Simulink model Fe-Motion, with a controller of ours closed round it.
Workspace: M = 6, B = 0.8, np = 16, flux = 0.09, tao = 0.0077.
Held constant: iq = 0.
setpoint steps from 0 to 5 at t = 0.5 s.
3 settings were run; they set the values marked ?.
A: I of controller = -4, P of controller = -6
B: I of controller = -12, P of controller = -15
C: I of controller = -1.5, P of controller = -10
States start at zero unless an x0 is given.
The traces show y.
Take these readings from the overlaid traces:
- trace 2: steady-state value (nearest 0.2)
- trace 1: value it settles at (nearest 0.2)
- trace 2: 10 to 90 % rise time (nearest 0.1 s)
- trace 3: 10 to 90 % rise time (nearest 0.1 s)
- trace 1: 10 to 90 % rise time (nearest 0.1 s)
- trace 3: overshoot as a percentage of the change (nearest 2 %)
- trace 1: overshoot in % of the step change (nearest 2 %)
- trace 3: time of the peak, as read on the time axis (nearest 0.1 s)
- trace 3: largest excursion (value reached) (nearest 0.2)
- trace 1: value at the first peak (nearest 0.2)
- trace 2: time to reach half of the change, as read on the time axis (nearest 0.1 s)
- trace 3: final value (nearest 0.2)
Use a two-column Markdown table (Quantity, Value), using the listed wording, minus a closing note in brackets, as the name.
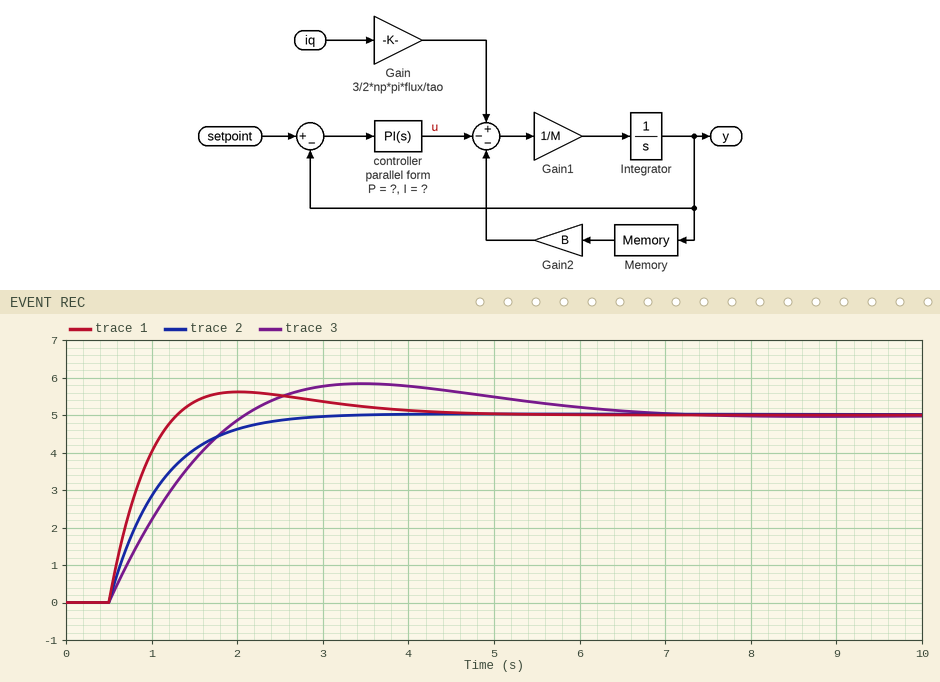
| Quantity | Value |
|---|---|
| trace 2: steady-state value | 5.0 |
| trace 1: value it settles at | 5.0 |
| trace 2: 10 to 90 % rise time | 1.3 s |
| trace 3: 10 to 90 % rise time | 1.2 s |
| trace 1: 10 to 90 % rise time | 0.6 s |
| trace 3: overshoot as a percentage of the change | 16 % |
| trace 1: overshoot in % of the step change | 12 % |
| trace 3: time of the peak, as read on the time axis | 3.5 s |
| trace 3: largest excursion (value reached) | 5.8 |
| trace 1: value at the first peak | 5.6 |
| trace 2: time to reach half of the change, as read on the time axis | 0.9 s |
| trace 3: final value | 5.0 |
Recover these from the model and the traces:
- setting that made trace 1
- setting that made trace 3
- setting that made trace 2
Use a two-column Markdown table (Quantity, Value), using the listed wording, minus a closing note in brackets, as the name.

| Quantity | Value |
|---|---|
| setting that made trace 1 | B |
| setting that made trace 3 | A |
| setting that made trace 2 | C |
